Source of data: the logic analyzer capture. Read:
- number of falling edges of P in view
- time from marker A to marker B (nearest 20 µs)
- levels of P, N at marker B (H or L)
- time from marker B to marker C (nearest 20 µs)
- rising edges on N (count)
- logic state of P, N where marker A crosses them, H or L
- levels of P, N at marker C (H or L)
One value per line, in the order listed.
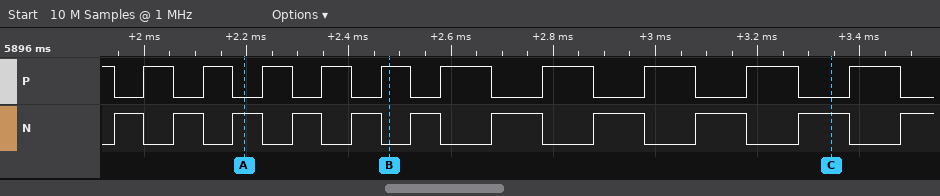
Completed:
11
280 µs
P=H, N=L
860 µs
11
P=L, N=H
P=L, N=H
